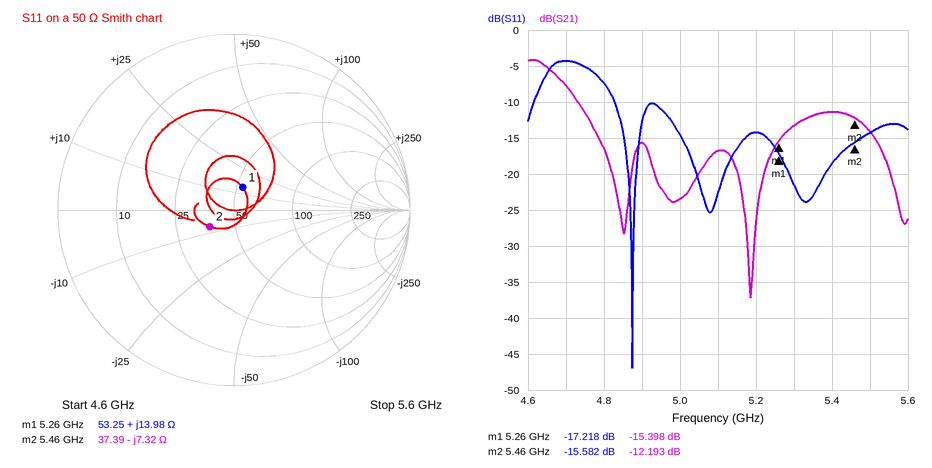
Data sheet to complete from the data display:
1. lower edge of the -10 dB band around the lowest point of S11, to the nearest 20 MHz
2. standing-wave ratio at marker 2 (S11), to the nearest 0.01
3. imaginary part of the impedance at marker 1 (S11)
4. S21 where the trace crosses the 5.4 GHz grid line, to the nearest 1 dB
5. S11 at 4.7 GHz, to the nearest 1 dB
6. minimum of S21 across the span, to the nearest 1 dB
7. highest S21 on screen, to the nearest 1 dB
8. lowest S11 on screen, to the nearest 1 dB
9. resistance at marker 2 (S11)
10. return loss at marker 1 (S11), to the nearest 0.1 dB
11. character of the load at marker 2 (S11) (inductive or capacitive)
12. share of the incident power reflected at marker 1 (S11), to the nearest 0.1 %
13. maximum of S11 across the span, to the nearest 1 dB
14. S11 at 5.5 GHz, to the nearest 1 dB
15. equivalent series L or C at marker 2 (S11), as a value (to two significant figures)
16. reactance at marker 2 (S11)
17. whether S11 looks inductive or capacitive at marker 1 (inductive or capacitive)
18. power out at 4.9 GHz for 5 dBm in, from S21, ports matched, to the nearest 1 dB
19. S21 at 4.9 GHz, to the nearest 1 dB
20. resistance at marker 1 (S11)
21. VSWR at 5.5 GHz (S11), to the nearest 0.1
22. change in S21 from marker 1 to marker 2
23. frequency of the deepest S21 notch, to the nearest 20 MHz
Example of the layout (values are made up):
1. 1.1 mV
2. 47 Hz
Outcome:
1. 4.82 GHz
2. 1.40
3. +13.98 Ω
4. -11 dB
5. -4 dB
6. -37 dB
7. -4 dB
8. -47 dB
9. 37.39 Ω
10. 17.2 dB
11. capacitive
12. 1.9 %
13. -4 dB
14. -14 dB
15. 4.0 pF
16. -7.32 Ω
17. inductive
18. -11 dBm
19. -16 dB
20. 53.25 Ω
21. 1.5
22. 3.205 dB
23. 5.18 GHz
